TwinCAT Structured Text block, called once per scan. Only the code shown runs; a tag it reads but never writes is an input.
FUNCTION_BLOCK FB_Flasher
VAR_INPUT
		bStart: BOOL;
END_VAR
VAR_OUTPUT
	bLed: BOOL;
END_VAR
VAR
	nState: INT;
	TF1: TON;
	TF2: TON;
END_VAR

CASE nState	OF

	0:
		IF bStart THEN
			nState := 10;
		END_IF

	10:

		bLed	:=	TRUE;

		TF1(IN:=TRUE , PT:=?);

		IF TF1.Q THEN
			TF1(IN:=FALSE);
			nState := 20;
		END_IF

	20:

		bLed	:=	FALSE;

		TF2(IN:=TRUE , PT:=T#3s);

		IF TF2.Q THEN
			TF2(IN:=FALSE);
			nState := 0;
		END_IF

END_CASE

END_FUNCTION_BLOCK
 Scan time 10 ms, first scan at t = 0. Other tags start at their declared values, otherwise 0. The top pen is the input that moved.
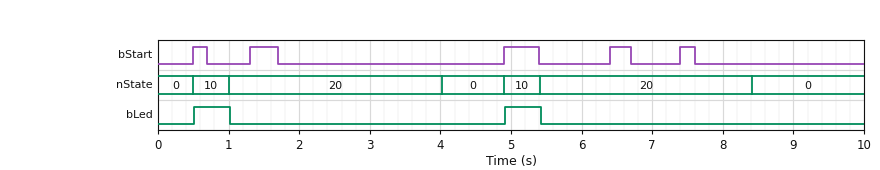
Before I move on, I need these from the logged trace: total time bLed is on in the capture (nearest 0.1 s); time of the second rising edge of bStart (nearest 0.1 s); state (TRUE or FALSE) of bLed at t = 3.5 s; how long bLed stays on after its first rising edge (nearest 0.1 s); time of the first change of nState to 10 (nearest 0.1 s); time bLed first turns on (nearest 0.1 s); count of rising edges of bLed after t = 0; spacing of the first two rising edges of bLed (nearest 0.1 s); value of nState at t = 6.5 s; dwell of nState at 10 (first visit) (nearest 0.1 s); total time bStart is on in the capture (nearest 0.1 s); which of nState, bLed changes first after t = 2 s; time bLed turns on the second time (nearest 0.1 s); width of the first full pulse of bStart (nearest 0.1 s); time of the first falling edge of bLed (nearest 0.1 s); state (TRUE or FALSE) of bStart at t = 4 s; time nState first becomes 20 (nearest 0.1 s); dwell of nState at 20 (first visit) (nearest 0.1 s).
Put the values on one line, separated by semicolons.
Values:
1.0 s; 1.3 s; FALSE; 0.5 s; 0.5 s; 0.5 s; 2; 4.4 s; 20; 0.5 s; 1.6 s; nState; 4.9 s; 0.2 s; 1.0 s; FALSE; 1.0 s; 3.0 s
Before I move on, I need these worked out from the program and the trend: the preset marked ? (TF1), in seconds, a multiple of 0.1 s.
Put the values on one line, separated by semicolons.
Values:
0.5 s
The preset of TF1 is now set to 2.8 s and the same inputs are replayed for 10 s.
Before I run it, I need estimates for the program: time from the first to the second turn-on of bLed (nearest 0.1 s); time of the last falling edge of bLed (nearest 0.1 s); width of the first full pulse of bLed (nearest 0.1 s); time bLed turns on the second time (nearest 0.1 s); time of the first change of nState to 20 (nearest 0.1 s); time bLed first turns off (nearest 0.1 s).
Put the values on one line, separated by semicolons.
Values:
5.9 s; 9.2 s; 2.8 s; 6.4 s; 3.3 s; 3.3 s
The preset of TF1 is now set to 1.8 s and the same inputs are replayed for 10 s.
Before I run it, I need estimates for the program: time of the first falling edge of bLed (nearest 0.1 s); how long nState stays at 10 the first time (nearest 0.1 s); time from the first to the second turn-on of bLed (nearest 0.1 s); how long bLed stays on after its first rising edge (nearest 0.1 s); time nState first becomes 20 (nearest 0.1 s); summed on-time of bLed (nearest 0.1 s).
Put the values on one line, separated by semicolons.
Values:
2.3 s; 1.8 s; 4.8 s; 1.8 s; 2.3 s; 3.6 s
